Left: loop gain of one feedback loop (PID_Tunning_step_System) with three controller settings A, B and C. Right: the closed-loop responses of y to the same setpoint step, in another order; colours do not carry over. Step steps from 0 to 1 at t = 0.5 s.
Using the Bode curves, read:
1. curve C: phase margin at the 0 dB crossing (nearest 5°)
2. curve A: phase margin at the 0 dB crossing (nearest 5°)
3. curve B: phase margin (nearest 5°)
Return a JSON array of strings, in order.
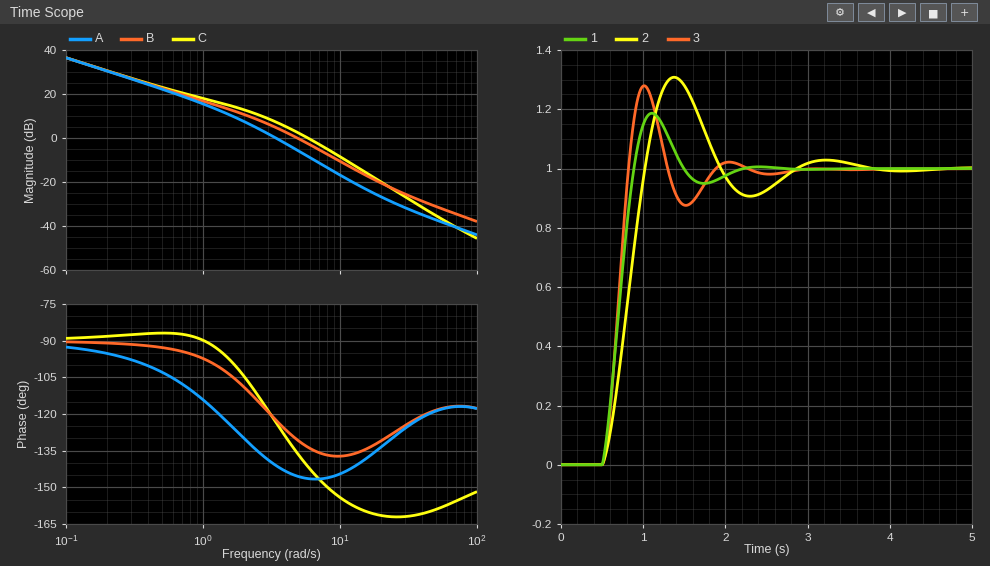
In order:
["40°", "40°", "50°"]
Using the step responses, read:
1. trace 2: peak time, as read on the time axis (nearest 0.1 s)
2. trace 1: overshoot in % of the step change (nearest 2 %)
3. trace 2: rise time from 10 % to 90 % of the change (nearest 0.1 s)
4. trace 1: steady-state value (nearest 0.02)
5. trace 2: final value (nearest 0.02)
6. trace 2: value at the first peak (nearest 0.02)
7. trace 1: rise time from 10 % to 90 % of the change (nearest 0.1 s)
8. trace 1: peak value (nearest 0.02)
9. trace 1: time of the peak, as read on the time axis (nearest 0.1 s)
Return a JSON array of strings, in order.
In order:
["1.4 s", "18 %", "0.4 s", "1.00", "1.00", "1.30", "0.3 s", "1.18", "1.1 s"]
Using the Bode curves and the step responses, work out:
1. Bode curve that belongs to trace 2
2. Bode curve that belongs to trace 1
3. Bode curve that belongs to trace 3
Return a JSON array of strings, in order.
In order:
["A", "B", "C"]
